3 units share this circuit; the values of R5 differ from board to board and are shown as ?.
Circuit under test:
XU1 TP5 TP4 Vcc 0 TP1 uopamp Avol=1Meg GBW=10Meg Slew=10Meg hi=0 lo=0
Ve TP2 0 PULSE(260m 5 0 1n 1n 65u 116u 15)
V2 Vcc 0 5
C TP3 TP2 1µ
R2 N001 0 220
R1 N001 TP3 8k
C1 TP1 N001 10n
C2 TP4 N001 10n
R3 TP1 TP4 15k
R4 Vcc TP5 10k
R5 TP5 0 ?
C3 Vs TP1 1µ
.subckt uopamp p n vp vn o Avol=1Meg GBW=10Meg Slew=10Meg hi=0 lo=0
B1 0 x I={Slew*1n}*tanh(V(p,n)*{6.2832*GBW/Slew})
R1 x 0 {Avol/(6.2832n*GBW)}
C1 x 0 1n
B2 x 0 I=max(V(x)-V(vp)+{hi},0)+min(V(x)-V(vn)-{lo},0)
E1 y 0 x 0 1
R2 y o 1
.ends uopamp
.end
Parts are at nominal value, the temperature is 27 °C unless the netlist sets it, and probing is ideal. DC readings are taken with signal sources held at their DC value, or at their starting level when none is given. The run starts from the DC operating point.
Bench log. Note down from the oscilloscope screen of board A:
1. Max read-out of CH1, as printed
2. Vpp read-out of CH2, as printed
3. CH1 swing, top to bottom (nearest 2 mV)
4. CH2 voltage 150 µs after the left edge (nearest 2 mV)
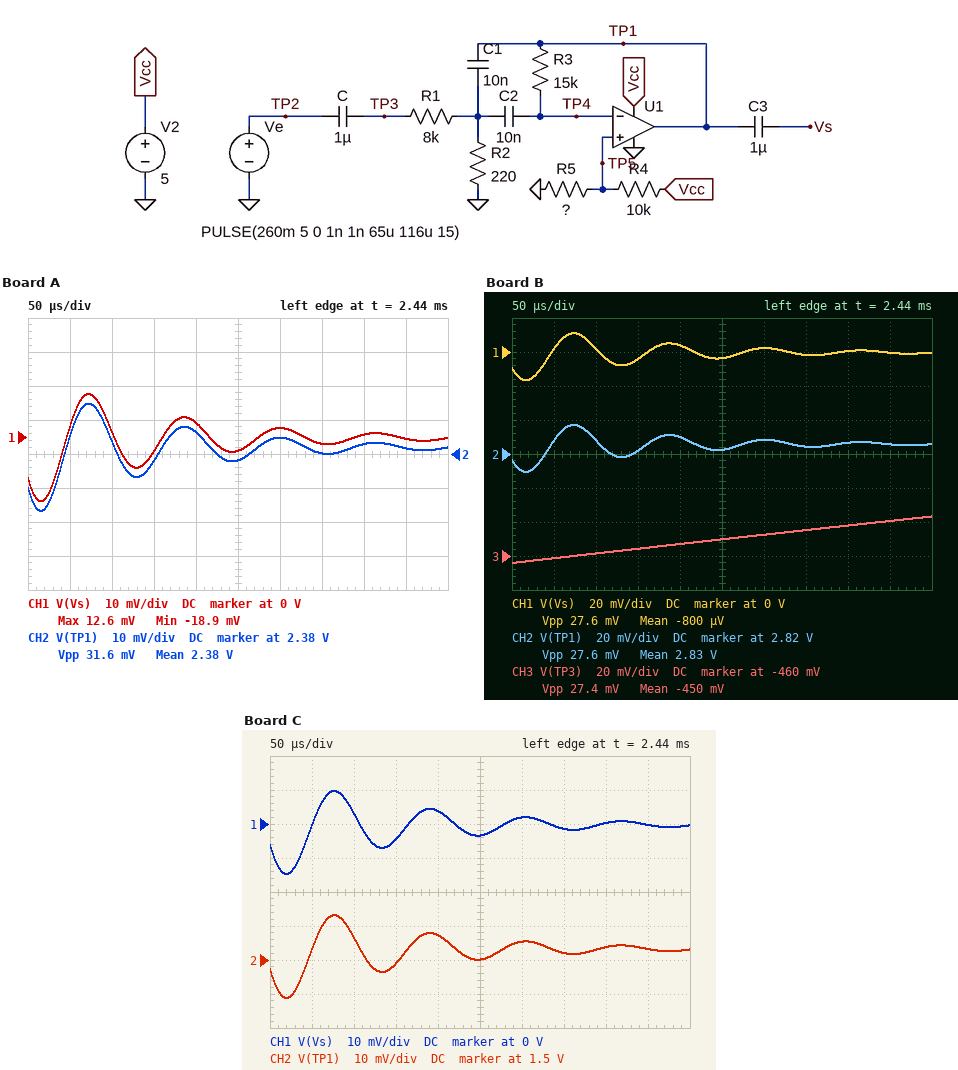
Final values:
12.6 mV
31.6 mV
32 mV
2.378 V
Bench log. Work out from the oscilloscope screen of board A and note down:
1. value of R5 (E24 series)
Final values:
9.1 kΩ
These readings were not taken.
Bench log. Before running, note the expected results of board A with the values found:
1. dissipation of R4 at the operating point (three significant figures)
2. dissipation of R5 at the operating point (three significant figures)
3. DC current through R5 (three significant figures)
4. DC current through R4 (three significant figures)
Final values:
685 µW
624 µW
262 µA
262 µA
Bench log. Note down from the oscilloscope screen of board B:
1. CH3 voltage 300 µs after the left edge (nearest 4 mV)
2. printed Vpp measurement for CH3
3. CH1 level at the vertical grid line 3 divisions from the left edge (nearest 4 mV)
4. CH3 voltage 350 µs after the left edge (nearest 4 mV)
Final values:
-448 mV
27.4 mV
-4 mV
-444 mV
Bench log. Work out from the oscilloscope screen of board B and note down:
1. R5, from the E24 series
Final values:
13 kΩ
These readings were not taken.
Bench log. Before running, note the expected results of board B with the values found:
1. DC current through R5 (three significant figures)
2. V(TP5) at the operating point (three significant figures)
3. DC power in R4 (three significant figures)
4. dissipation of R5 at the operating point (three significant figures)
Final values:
217 µA
2.83 V
473 µW
614 µW
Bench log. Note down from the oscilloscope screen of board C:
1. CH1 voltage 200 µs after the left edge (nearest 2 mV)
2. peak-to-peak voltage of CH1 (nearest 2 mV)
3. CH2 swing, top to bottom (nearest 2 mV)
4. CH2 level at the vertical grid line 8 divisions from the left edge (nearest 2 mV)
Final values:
4 mV
24 mV
24 mV
1.504 V
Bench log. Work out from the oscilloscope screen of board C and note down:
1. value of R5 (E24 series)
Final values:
4.3 kΩ
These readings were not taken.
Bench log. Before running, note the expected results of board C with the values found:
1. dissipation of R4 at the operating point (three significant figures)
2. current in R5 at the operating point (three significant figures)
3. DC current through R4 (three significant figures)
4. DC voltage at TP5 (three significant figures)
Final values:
1.22 mW
350 µA
350 µA
1.50 V
